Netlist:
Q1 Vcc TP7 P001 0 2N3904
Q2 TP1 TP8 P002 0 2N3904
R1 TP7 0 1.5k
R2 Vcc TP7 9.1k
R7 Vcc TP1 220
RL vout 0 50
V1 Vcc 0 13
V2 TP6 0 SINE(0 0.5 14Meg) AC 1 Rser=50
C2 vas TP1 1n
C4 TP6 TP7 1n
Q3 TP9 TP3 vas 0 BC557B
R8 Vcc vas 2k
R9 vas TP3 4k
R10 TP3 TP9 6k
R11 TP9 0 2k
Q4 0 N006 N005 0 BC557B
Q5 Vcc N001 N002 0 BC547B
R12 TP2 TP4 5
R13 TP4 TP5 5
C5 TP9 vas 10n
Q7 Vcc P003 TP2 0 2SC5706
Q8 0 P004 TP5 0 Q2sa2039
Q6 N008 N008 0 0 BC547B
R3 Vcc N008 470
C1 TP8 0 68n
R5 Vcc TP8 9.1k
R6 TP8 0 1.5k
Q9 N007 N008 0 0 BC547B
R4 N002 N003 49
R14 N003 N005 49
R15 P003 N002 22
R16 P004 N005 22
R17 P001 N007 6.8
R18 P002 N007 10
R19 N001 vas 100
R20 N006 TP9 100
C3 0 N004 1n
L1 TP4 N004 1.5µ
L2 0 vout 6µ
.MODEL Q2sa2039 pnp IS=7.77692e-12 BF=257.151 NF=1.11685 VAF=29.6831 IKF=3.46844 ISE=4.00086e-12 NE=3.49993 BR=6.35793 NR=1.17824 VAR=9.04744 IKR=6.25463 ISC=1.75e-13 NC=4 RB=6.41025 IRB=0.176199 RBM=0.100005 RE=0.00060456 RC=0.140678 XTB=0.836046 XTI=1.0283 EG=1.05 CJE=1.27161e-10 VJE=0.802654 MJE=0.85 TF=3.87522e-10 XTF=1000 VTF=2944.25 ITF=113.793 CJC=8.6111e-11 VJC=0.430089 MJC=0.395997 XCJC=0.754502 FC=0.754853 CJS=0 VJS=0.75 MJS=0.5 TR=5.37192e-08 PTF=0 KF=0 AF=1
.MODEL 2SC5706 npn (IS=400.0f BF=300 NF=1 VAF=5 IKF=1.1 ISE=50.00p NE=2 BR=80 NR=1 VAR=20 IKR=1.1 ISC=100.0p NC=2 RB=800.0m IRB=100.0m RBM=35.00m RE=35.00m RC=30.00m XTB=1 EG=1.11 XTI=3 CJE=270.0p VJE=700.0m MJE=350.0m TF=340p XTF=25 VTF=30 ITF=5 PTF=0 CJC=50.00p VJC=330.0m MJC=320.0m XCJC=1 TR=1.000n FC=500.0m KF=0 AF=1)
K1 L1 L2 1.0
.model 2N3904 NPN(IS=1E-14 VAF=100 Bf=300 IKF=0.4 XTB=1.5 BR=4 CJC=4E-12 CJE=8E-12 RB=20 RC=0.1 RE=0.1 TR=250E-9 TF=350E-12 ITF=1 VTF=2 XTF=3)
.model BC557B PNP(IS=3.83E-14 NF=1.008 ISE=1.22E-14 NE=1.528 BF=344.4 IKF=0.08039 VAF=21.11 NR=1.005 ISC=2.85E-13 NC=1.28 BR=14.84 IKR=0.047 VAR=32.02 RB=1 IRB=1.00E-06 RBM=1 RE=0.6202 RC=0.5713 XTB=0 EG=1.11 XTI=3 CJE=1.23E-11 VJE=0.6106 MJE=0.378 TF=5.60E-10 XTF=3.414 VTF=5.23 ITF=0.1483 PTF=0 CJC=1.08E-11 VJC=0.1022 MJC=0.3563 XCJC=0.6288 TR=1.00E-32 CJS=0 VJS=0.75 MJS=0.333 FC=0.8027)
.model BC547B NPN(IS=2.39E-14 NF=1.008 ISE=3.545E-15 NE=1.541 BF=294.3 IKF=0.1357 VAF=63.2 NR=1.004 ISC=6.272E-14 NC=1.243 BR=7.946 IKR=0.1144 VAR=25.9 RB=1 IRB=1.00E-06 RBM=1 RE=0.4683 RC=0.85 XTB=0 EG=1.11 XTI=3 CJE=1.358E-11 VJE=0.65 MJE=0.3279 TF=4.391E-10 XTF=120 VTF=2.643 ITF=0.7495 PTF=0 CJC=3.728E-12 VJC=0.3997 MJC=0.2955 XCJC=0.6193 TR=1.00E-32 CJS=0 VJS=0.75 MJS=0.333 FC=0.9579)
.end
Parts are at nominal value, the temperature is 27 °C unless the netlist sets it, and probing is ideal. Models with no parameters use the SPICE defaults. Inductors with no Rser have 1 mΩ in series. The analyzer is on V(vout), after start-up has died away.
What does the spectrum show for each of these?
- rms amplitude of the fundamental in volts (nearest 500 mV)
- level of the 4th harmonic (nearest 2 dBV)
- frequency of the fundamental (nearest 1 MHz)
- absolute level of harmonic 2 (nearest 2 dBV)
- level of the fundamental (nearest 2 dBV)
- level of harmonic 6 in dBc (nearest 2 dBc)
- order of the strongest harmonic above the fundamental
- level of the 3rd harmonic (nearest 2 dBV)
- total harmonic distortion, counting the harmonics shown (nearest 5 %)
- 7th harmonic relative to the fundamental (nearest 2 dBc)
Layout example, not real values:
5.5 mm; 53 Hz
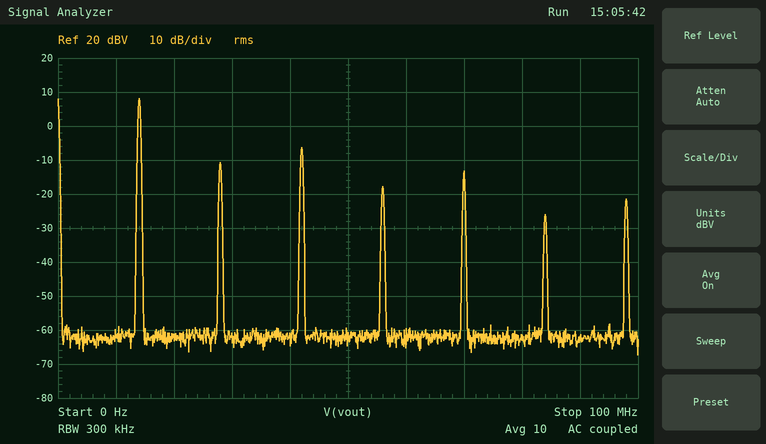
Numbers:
2.5 V; -18 dBV; 14 MHz; -10 dBV; 8 dBV; -34 dBc; 3; -6 dBV; 25 %; -30 dBc
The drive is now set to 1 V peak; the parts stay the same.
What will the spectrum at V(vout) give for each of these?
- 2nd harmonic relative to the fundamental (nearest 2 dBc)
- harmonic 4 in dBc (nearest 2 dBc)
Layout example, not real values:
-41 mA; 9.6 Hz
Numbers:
-22 dBc; -30 dBc
